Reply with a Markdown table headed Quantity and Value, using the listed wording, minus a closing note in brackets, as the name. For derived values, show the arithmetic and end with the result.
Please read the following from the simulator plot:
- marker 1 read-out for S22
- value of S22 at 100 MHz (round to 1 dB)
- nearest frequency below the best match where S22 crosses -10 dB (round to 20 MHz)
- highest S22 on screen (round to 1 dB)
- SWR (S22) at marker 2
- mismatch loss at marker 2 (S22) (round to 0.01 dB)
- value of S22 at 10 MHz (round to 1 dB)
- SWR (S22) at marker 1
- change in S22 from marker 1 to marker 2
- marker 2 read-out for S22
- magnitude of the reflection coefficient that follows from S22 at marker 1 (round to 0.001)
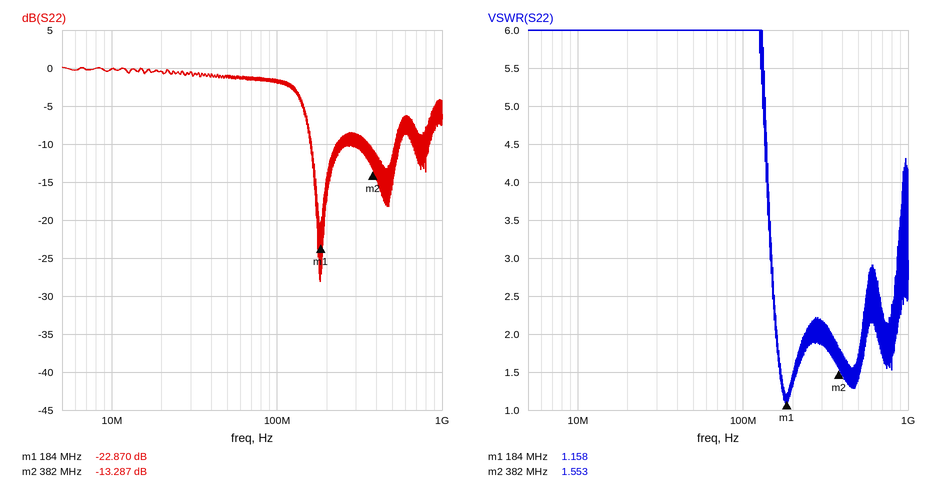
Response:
| Quantity | Value |
|---|---|
| marker 1 read-out for S22 | -22.870 dB |
| value of S22 at 100 MHz | -2 dB |
| nearest frequency below the best match where S22 crosses -10 dB | 160 MHz |
| highest S22 on screen | 0 dB |
| SWR (S22) at marker 2 | 1.553 |
| mismatch loss at marker 2 (S22) | −10 log10(1 − 10^(-13.287/10)) ≈ 0.21 dB |
| value of S22 at 10 MHz | 0 dB |
| SWR (S22) at marker 1 | 1.158 |
| change in S22 from marker 1 to marker 2 | -13.287 − (-22.87) = 9.583 dB |
| marker 2 read-out for S22 | -13.287 dB |
| magnitude of the reflection coefficient that follows from S22 at marker 1 | 10^(-22.87/20) ≈ 0.072 |
